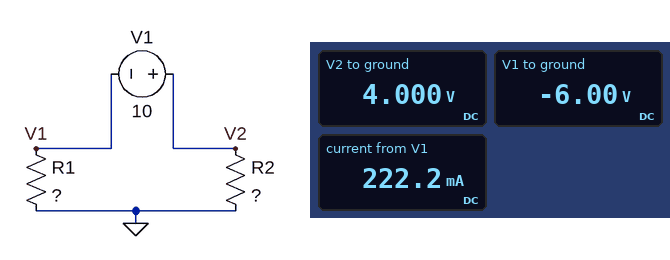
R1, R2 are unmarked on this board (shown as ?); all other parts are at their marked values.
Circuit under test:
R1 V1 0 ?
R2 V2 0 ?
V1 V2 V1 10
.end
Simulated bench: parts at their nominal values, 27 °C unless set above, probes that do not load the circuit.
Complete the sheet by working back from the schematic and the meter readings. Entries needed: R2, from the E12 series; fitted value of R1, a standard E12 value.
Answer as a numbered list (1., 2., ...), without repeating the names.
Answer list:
1. 18 Ω
2. 27 Ω
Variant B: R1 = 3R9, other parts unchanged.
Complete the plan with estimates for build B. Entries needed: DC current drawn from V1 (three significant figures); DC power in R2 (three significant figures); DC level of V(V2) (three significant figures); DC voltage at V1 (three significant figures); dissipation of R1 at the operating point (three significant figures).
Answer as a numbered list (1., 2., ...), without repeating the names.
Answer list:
1. 457 mA
2. 3.75 W
3. 8.22 V
4. -1.78 V
5. 813 mW
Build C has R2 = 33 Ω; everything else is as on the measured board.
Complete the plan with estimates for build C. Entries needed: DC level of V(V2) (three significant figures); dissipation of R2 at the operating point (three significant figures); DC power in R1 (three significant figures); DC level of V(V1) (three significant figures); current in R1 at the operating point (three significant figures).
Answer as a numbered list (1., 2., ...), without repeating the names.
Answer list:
1. 5.50 V
2. 917 mW
3. 750 mW
4. -4.50 V
5. 167 mA
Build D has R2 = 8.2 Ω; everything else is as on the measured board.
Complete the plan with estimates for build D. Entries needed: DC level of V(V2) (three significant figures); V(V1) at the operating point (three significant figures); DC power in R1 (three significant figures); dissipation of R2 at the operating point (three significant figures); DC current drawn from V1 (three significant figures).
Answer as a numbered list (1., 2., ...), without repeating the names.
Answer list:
1. 2.33 V
2. -7.67 V
3. 2.18 W
4. 662 mW
5. 284 mA
